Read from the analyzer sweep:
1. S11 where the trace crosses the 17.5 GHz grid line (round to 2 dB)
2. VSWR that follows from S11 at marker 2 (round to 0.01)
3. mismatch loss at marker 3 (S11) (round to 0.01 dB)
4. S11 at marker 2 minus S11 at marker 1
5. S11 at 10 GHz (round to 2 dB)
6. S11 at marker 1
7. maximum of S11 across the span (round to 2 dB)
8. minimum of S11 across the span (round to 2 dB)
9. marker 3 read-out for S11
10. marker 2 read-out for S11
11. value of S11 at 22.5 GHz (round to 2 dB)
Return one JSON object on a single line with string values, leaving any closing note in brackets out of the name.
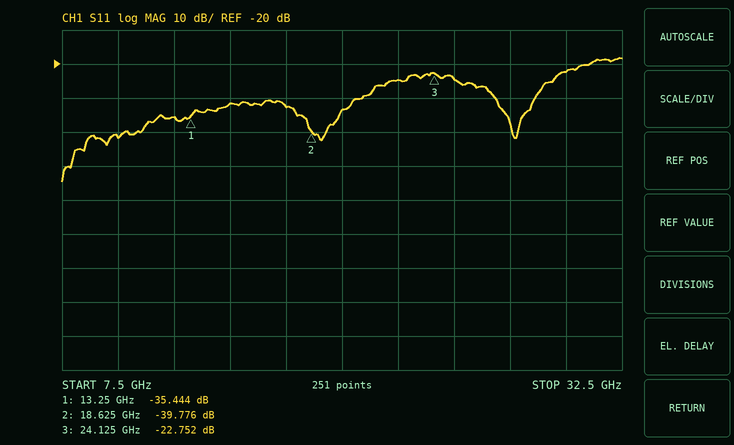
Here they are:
{"S11 where the trace crosses the 17.5 GHz grid line": "-32 dB", "VSWR that follows from S11 at marker 2": "1.02", "mismatch loss at marker 3 (S11)": "0.02 dB", "S11 at marker 2 minus S11 at marker 1": "-4.332 dB", "S11 at 10 GHz": "-42 dB", "S11 at marker 1": "-35.444 dB", "maximum of S11 across the span": "-18 dB", "minimum of S11 across the span": "-54 dB", "marker 3 read-out for S11": "-22.752 dB", "marker 2 read-out for S11": "-39.776 dB", "value of S11 at 22.5 GHz": "-24 dB"}
